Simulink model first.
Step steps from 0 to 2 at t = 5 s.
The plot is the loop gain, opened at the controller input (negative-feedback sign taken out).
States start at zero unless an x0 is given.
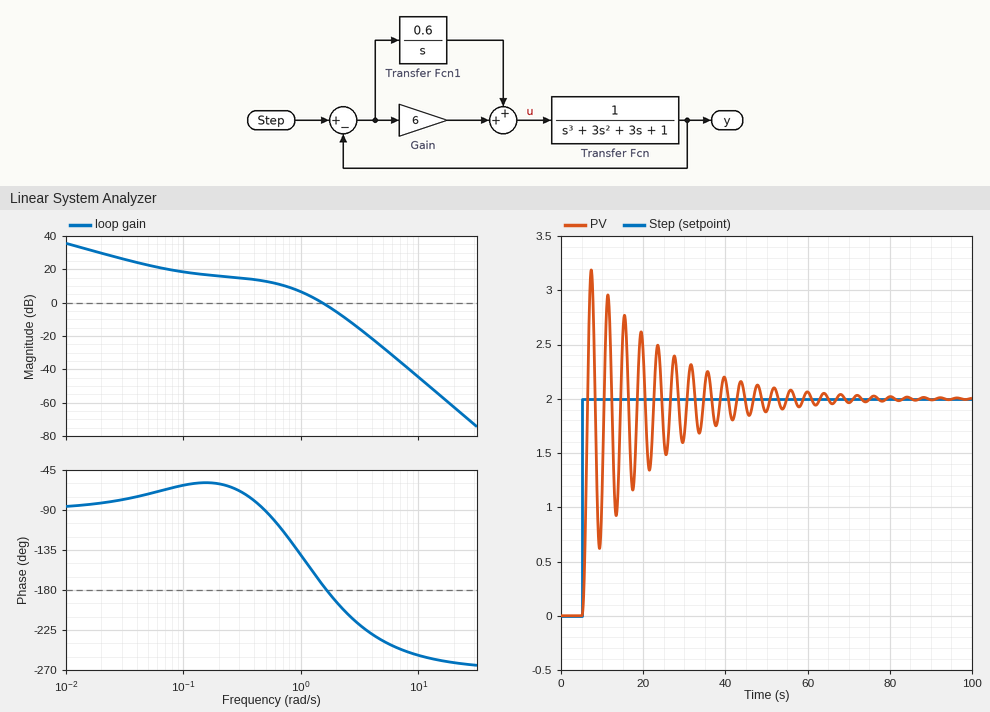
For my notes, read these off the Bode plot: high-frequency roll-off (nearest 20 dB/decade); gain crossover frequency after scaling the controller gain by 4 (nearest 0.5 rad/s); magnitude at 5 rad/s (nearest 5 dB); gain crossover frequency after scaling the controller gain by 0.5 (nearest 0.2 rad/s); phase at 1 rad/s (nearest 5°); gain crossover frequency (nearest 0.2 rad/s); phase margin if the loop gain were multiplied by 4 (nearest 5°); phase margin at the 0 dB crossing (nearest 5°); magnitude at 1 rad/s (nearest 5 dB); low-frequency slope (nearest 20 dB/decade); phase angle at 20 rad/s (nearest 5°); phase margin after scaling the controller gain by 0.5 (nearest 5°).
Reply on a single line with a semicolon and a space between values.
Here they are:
-60 dB/decade; 2.5 rad/s; -25 dB; 1.0 rad/s; -140°; 1.6 rad/s; -30°; 5°; 5 dB; -20 dB/decade; -260°; 35°
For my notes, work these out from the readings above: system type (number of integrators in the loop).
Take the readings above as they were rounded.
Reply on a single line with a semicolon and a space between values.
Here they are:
1
